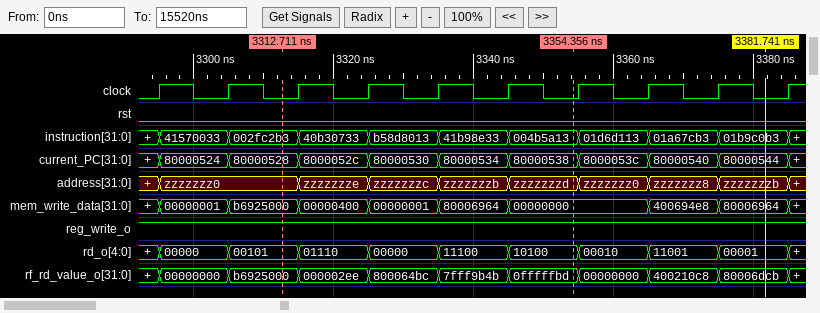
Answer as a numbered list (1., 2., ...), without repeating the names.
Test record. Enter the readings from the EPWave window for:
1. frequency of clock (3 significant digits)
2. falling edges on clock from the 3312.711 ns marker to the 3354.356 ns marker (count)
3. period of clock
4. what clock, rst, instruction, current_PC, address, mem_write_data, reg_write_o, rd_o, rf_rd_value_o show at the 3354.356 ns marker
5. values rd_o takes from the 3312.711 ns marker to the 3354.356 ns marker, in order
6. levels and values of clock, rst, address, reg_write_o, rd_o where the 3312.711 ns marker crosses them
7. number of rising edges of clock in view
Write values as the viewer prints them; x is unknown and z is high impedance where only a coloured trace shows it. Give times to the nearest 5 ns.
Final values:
1. 100 MHz
2. 4
3. 10 ns
4. clock=0, rst=0, instruction=004b5a13, current_PC=80000538, address=zzzzzzzd, mem_write_data=00000000, reg_write_o=1, rd_o=10100, rf_rd_value_o=0fffffbd
5. 00101, 01110, 00000, 11100, 10100
6. clock=0, rst=0, address=zzzzzzz0, reg_write_o=1, rd_o=00101
7. 10
